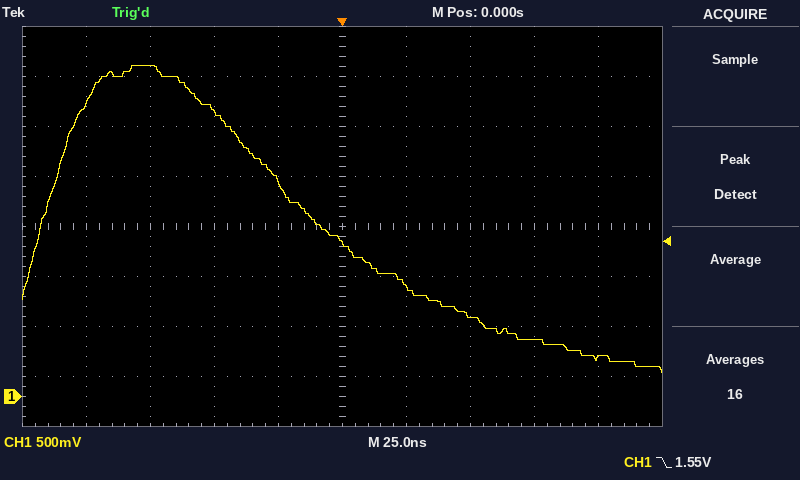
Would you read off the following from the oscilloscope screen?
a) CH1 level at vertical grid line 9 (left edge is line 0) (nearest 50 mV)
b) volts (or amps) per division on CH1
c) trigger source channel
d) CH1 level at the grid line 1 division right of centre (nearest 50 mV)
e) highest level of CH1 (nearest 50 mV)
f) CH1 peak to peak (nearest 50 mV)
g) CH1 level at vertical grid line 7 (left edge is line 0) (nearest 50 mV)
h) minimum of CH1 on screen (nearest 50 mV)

400 mV
500 mV
CH1
1.10 V
3.30 V
3.05 V
800 mV
250 mV
